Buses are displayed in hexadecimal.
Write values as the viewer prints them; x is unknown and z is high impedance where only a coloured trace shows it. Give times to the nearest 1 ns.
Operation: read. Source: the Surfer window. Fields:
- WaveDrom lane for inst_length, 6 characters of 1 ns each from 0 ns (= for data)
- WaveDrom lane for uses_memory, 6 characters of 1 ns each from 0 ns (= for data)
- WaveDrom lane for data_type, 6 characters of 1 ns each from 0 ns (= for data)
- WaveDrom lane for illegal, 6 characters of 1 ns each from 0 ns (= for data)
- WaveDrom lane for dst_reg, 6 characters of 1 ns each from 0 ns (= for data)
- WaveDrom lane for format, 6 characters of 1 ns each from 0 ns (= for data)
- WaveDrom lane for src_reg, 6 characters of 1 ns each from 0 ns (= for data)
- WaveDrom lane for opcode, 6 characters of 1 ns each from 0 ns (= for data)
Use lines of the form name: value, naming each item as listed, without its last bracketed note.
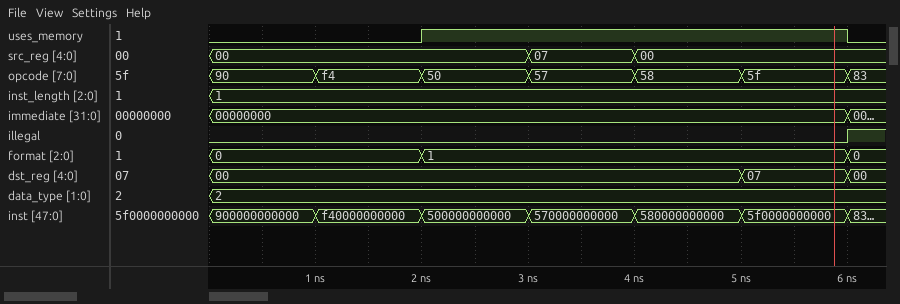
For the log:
WaveDrom lane for inst_length, 6 characters of 1 ns each from 0 ns: {name: 'inst_length', wave: '=.....', data: '1'}
WaveDrom lane for uses_memory, 6 characters of 1 ns each from 0 ns: {name: 'uses_memory', wave: '0.1...'}
WaveDrom lane for data_type, 6 characters of 1 ns each from 0 ns: {name: 'data_type', wave: '=.....', data: '2'}
WaveDrom lane for illegal, 6 characters of 1 ns each from 0 ns: {name: 'illegal', wave: '0.....'}
WaveDrom lane for dst_reg, 6 characters of 1 ns each from 0 ns: {name: 'dst_reg', wave: '=....=', data: '00 07'}
WaveDrom lane for format, 6 characters of 1 ns each from 0 ns: {name: 'format', wave: '=.=...', data: '0 1'}
WaveDrom lane for src_reg, 6 characters of 1 ns each from 0 ns: {name: 'src_reg', wave: '=..==.', data: '00 07 00'}
WaveDrom lane for opcode, 6 characters of 1 ns each from 0 ns: {name: 'opcode', wave: '======', data: '90 f4 50 57 58 5f'}
